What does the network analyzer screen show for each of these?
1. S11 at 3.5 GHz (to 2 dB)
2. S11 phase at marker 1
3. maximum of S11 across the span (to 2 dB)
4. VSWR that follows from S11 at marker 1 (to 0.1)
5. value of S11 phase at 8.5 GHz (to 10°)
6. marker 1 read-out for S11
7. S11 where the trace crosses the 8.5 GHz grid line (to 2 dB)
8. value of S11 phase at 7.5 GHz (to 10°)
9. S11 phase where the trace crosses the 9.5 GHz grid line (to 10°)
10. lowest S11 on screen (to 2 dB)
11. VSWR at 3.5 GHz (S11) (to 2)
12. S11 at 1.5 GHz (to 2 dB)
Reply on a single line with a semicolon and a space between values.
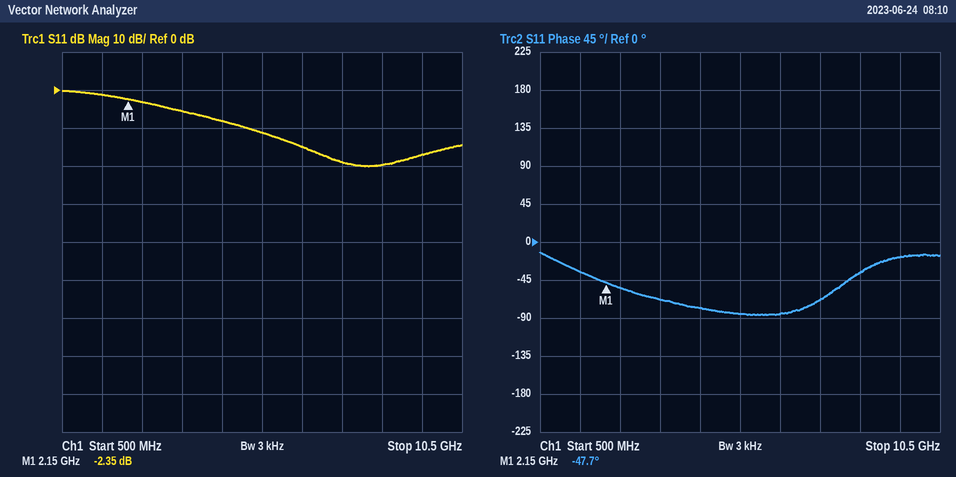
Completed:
-6 dB; -47.7°; 0 dB; 7.4; -40°; -2.35 dB; -20 dB; -70°; -20°; -20 dB; 4; -2 dB
